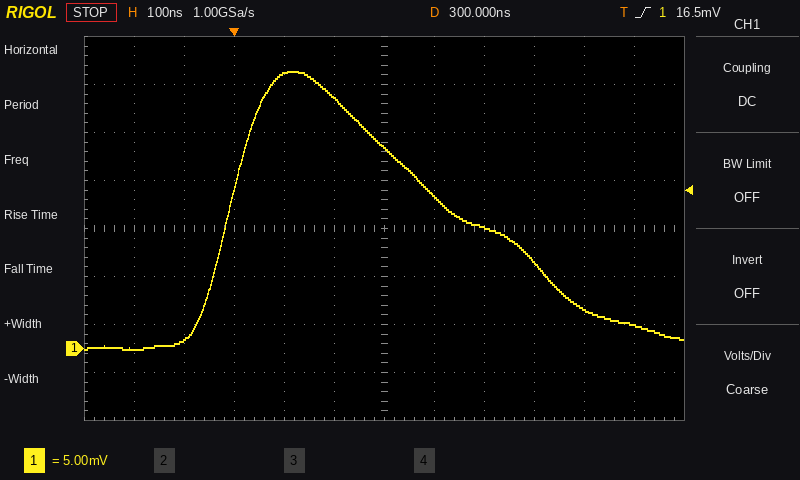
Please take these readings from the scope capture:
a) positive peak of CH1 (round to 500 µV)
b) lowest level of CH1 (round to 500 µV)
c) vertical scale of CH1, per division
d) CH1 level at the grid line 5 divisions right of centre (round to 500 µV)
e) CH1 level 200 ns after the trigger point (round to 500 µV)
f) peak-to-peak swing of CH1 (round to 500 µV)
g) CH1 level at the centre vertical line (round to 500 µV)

29.0 mV
0.0 mV
5 mV
2.5 mV
26.0 mV
29.0 mV
21.0 mV
